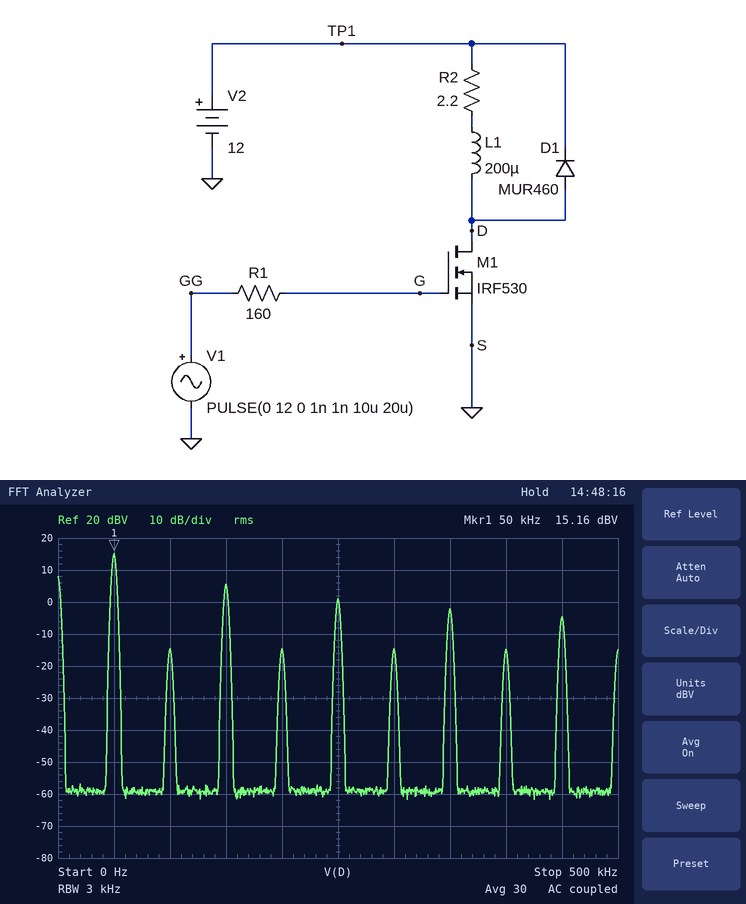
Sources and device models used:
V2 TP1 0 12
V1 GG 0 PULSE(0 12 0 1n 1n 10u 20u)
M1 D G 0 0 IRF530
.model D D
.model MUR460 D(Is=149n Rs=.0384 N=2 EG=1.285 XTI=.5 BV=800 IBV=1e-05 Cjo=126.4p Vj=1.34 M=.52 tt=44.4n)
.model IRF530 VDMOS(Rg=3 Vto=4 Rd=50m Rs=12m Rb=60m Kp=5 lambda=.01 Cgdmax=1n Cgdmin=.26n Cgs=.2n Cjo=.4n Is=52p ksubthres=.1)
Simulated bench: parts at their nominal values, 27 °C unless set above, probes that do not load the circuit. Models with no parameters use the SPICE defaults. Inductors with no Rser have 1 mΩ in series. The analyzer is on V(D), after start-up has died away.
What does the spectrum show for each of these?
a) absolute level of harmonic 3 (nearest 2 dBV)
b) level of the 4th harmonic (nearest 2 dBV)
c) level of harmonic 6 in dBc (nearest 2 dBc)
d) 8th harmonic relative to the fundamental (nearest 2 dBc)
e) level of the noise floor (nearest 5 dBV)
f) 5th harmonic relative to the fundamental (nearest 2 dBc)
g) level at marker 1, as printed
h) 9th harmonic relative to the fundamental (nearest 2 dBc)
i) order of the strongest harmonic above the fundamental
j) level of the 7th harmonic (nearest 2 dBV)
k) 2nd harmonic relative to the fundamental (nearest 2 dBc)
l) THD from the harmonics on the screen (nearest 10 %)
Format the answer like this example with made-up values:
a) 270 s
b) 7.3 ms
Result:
a) 6 dBV
b) -14 dBV
c) -30 dBc
d) -30 dBc
e) -60 dBV
f) -14 dBc
g) 15.16 dBV
h) -20 dBc
i) 3
j) -2 dBV
k) -30 dBc
l) 40 %
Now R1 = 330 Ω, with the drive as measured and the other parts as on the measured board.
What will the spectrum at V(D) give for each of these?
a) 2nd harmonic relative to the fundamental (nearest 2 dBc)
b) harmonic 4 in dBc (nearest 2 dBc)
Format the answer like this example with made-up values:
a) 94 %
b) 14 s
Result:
a) -24 dBc
b) -24 dBc
